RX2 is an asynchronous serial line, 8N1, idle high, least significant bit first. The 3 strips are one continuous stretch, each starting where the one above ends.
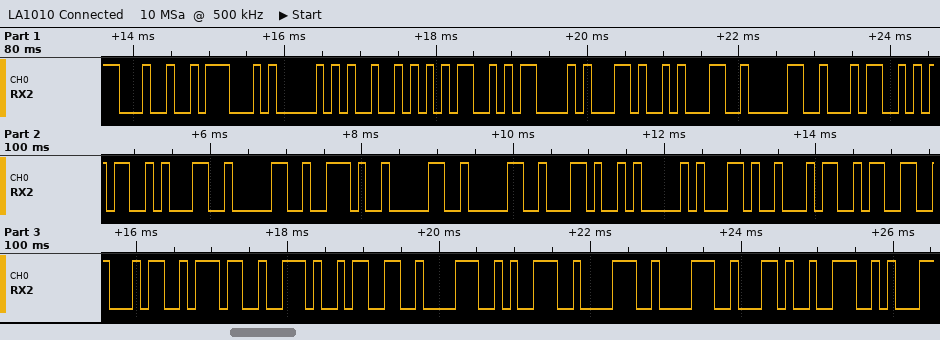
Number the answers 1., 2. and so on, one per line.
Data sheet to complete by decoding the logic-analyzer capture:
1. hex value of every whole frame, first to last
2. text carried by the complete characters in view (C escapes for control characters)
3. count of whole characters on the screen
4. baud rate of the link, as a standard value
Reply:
1. 24 47 50 52 4D 43 2C 31 30 34 35 31 30 2E 30 30 2C 41 2C 34 33 34 37 2E 33 38 39 38 38 2C 4E
2. "$GPRMC,104510.00,A,4347.38988,N"
3. 31
4. 9600 baud
